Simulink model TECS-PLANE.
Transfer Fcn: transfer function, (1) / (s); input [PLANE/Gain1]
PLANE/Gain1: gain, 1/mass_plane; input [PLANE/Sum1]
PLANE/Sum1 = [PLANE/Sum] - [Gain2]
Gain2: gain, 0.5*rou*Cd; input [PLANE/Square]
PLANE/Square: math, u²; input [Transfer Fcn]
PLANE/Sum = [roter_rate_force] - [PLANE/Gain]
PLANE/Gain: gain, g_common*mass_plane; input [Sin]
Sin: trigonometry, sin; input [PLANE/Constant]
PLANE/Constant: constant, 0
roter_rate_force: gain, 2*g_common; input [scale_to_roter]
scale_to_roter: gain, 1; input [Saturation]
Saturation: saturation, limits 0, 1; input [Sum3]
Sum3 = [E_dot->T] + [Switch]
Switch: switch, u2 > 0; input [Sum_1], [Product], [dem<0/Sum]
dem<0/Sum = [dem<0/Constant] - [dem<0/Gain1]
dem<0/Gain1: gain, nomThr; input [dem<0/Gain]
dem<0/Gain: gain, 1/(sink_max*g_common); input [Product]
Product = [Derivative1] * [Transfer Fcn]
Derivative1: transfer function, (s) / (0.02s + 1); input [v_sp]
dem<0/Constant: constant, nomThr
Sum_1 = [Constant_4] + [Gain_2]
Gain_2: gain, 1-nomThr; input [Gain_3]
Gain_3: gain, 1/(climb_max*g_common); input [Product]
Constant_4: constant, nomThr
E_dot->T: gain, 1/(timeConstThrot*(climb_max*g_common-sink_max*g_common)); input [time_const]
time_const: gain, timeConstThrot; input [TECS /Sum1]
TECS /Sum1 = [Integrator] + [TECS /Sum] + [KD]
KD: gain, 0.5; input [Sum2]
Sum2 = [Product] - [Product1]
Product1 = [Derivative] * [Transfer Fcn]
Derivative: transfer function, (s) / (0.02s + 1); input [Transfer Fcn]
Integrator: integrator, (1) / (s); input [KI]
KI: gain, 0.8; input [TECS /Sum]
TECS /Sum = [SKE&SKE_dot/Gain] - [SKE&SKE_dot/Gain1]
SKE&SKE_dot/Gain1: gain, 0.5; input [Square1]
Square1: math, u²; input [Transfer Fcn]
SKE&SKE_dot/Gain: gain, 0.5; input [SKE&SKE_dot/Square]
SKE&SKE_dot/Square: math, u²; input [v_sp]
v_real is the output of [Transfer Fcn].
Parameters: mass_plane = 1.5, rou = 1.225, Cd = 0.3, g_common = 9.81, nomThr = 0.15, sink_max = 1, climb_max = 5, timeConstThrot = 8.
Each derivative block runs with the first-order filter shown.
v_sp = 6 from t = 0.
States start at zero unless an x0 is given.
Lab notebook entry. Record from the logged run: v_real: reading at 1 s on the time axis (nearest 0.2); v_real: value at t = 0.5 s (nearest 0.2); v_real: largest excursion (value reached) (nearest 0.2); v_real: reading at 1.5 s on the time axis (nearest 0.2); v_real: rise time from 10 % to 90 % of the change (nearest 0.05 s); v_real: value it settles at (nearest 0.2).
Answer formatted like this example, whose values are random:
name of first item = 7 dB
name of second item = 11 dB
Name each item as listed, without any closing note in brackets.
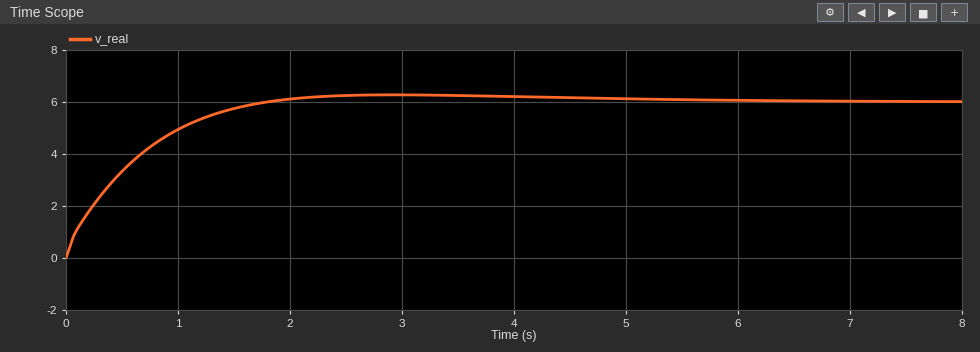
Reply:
v_real: reading at 1 s on the time axis = 5.0
v_real: value at t = 0.5 s = 3.4
v_real: largest excursion (value reached) = 6.2
v_real: reading at 1.5 s on the time axis = 5.8
v_real: rise time from 10 % to 90 % of the change = 1.20 s
v_real: value it settles at = 6.0
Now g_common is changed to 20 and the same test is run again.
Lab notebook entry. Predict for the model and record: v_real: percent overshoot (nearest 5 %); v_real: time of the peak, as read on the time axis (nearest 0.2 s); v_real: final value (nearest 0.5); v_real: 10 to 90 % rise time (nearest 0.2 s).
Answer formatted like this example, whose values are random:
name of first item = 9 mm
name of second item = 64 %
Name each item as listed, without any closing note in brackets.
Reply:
v_real: percent overshoot = 10 %
v_real: time of the peak, as read on the time axis = 2.4 s
v_real: final value = 6.0
v_real: 10 to 90 % rise time = 1.0 s
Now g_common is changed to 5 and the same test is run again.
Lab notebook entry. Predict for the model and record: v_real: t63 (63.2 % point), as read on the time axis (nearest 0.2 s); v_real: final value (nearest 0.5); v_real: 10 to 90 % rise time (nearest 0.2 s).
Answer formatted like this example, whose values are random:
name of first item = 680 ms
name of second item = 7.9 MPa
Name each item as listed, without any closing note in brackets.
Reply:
v_real: t63 (63.2 % point), as read on the time axis = 0.8 s
v_real: final value = 6.0
v_real: 10 to 90 % rise time = 1.4 s
